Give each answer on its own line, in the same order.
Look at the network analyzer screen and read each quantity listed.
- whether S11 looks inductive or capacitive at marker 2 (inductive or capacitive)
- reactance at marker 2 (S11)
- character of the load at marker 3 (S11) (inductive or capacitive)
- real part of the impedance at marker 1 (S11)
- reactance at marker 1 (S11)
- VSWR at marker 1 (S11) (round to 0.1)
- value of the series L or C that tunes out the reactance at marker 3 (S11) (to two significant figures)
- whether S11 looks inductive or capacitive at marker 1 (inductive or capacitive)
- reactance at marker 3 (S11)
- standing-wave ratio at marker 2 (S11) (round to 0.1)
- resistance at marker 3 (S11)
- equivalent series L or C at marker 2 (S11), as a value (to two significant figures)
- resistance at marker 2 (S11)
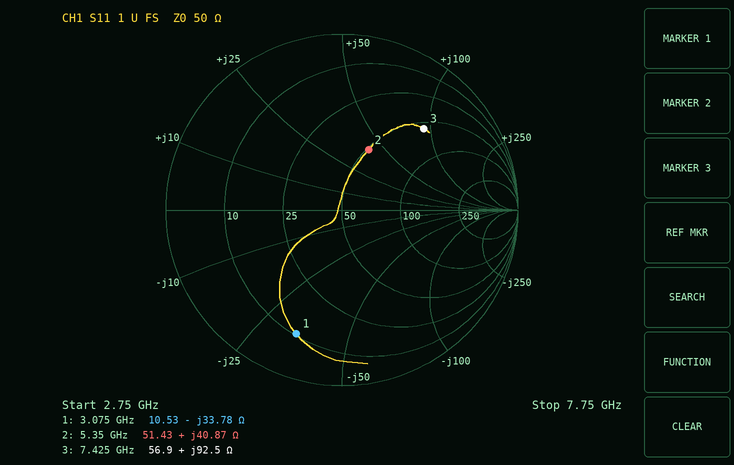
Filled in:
inductive
+40.87 Ω
inductive
10.53 Ω
-33.78 Ω
7.0
230 fF
capacitive
+92.5 Ω
2.2
56.9 Ω
1.2 nH
51.43 Ω
